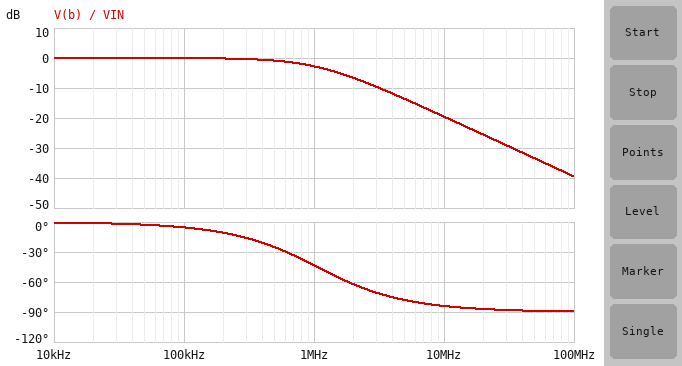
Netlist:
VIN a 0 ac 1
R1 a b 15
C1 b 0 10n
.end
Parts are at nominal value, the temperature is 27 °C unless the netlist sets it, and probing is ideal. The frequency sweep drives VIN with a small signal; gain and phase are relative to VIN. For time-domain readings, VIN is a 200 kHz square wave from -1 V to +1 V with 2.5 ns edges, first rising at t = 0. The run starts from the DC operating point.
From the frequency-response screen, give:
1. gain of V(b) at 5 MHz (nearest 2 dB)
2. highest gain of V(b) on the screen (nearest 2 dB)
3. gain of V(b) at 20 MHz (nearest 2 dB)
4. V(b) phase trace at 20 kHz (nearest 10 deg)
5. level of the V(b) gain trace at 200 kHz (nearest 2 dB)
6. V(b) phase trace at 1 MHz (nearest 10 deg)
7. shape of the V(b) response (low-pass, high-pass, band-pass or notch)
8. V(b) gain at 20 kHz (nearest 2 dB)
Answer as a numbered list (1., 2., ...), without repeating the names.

1. -14 dB
2. 0 dB
3. -26 dB
4. 0 deg
5. 0 dB
6. -40 deg
7. low-pass
8. 0 dB
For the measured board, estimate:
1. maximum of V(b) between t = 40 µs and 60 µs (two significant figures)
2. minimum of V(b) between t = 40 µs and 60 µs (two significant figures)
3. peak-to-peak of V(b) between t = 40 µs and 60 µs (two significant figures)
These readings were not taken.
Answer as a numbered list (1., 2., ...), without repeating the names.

1. 1.0 V
2. -1.0 V
3. 2.0 V
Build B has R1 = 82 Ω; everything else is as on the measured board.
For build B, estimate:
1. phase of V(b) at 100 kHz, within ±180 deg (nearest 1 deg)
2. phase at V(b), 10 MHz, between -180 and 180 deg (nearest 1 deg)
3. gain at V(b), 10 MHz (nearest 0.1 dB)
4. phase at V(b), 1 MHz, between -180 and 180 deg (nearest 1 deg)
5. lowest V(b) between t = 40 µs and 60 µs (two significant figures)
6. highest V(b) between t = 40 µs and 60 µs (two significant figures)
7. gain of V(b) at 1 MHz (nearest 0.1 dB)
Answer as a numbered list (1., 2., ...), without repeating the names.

1. -27 deg
2. -89 deg
3. -34.2 dB
4. -79 deg
5. -910 mV
6. 910 mV
7. -14.4 dB
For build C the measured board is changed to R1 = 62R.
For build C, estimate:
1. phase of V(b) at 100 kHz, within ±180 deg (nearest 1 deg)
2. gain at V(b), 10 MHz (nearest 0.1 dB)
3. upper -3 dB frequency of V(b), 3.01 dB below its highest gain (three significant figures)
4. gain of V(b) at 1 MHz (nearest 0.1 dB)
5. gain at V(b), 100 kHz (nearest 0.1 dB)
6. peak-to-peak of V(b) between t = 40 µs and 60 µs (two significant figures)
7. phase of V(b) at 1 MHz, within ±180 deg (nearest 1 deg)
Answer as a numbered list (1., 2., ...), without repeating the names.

1. -21 deg
2. -31.8 dB
3. 257 kHz
4. -12.1 dB
5. -0.6 dB
6. 1.9 V
7. -76 deg
